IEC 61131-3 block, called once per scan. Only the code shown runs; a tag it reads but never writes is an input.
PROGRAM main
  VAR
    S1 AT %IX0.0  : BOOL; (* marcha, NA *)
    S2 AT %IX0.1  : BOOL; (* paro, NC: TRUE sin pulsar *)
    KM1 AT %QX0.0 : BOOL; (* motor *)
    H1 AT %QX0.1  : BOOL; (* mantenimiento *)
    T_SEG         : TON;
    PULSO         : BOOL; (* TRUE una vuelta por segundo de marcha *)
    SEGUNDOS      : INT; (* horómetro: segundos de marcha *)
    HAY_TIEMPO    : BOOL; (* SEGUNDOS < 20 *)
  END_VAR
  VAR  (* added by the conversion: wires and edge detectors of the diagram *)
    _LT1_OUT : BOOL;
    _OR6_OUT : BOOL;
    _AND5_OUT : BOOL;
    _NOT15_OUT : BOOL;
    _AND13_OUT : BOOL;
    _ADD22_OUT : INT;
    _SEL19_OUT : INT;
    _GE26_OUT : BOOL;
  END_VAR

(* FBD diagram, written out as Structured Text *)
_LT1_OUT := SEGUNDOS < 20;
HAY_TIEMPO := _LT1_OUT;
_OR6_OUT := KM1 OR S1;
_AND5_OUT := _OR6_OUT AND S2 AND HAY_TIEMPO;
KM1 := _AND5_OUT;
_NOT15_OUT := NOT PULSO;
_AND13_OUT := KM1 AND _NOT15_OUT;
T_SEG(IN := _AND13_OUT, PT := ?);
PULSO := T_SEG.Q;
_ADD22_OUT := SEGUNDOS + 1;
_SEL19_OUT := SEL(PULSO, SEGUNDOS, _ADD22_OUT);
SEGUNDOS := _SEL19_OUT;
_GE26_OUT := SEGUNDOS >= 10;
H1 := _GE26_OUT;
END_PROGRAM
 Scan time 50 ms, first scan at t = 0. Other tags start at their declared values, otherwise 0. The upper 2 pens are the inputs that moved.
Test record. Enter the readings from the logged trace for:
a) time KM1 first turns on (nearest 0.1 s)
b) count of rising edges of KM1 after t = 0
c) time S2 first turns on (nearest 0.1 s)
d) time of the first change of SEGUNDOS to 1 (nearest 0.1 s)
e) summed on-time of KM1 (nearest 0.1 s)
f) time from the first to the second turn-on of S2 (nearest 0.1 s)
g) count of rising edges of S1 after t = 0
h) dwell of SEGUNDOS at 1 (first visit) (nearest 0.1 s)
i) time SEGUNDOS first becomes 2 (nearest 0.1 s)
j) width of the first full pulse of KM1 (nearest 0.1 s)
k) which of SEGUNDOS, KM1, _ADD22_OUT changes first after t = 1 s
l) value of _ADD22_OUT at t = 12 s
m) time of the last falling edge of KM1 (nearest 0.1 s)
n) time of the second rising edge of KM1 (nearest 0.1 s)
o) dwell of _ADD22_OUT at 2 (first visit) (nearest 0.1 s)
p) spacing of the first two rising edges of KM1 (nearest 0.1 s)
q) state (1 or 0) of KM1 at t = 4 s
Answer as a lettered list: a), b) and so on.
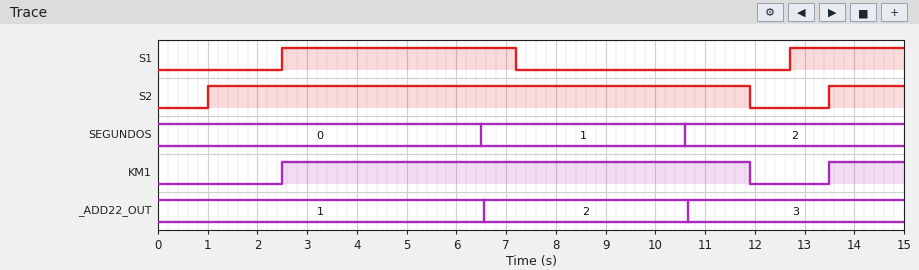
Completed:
a) 2.5 s
b) 2
c) 1.0 s
d) 6.5 s
e) 10.9 s
f) 12.5 s
g) 2
h) 4.1 s
i) 10.6 s
j) 9.4 s
k) KM1
l) 3
m) 11.9 s
n) 13.5 s
o) 4.1 s
p) 11.0 s
q) 1
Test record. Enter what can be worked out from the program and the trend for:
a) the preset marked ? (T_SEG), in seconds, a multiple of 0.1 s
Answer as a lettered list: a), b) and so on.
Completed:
a) 4.0 s
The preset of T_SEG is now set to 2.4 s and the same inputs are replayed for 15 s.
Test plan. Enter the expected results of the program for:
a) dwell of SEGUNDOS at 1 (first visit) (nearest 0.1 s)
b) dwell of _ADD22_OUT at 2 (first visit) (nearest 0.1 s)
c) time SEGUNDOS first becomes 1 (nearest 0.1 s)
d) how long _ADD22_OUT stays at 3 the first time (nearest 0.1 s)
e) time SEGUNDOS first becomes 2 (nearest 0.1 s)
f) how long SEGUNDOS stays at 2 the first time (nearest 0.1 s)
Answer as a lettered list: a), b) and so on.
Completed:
a) 2.5 s
b) 2.5 s
c) 4.9 s
d) 2.5 s
e) 7.4 s
f) 2.5 s
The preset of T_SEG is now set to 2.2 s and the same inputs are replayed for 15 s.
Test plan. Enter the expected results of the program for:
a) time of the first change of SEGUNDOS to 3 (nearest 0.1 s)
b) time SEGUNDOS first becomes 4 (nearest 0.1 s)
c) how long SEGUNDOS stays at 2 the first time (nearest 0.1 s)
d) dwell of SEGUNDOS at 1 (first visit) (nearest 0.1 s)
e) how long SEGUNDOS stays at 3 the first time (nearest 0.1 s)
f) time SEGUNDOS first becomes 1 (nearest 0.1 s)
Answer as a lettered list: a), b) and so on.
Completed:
a) 9.3 s
b) 11.6 s
c) 2.3 s
d) 2.3 s
e) 2.3 s
f) 4.7 s
